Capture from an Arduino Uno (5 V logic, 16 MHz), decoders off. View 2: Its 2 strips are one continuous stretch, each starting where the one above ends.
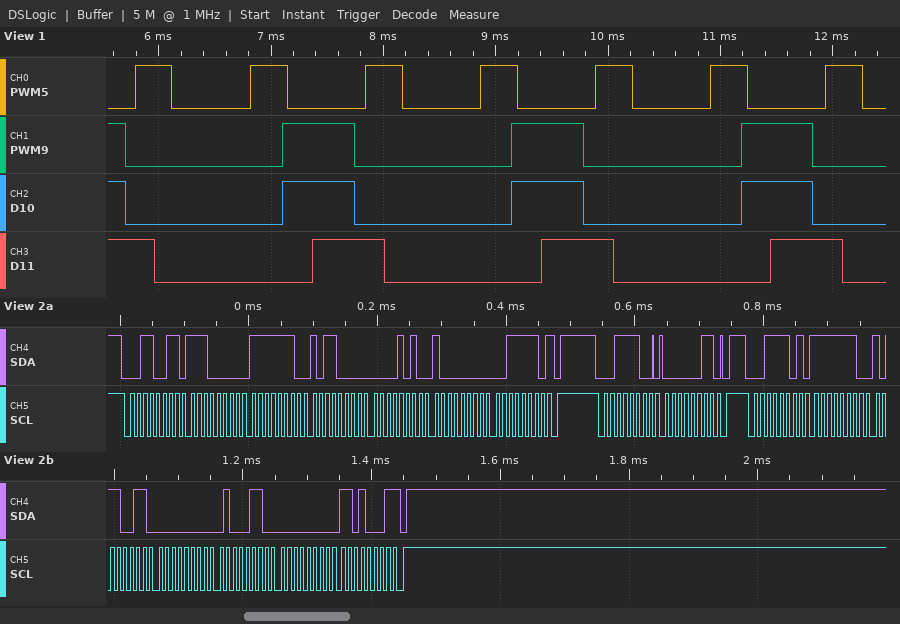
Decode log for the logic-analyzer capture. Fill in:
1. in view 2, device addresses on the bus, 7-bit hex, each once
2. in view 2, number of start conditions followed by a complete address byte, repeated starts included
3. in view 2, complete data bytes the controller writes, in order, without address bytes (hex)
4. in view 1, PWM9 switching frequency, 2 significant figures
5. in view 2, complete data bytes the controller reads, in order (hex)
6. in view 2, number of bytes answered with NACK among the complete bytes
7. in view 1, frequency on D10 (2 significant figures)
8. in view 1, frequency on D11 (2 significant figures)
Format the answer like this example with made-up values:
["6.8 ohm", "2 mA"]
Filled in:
["0x19 0x1E", "3", "03", "490 Hz", "E0 FE B0 0A 80 3E FE B3 00 46 00 D1", "2", "490 Hz", "490 Hz"]
